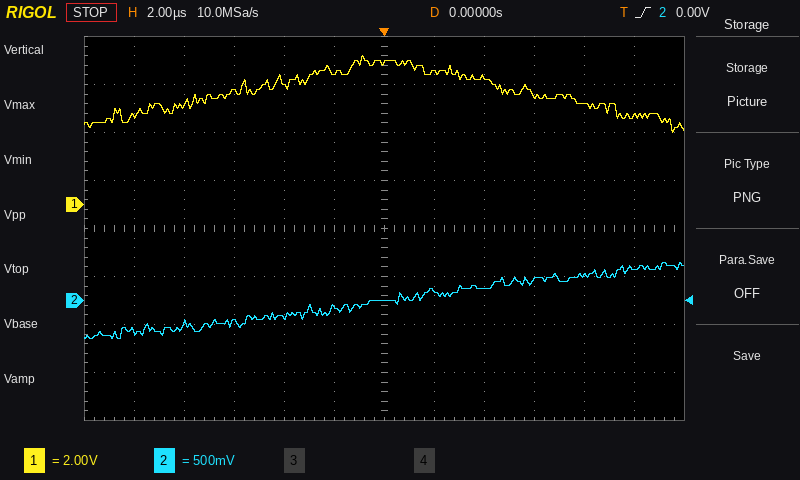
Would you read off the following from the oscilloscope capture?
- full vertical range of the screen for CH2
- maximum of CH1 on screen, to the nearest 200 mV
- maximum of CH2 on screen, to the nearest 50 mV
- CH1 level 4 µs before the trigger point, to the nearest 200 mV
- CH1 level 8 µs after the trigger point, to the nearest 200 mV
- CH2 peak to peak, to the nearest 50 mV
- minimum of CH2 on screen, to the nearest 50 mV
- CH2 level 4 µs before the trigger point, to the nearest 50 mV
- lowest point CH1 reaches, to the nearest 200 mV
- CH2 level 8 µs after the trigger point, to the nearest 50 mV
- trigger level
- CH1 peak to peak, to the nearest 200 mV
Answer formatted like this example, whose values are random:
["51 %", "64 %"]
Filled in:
["4 V", "6.2 V", "400 mV", "5.0 V", "4.2 V", "800 mV", "-400 mV", "-150 mV", "3.0 V", "250 mV", "0.00 V", "3.2 V"]
